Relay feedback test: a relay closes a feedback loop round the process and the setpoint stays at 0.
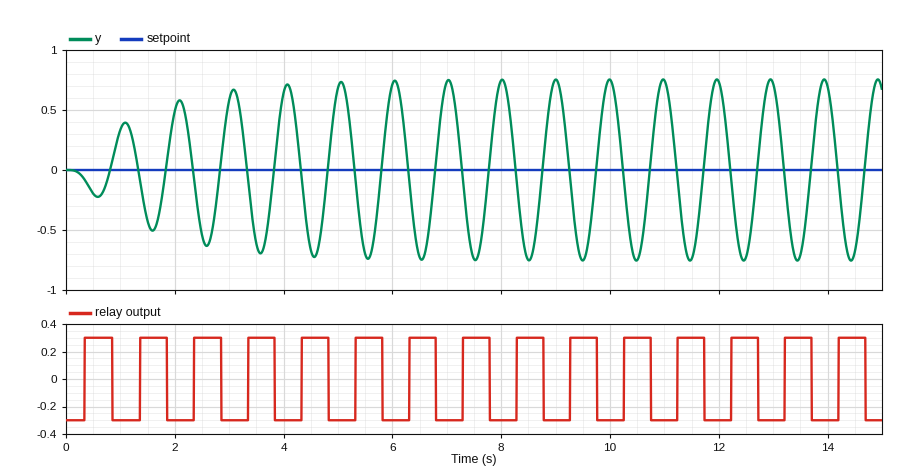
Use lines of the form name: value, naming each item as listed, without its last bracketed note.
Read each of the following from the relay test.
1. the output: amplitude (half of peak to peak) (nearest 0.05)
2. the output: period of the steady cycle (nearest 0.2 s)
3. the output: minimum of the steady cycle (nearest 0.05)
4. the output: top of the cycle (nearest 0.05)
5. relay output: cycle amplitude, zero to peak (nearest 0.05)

the output: amplitude (half of peak to peak): 0.75
the output: period of the steady cycle: 1.0 s
the output: minimum of the steady cycle: -0.75
the output: top of the cycle: 0.75
relay output: cycle amplitude, zero to peak: 0.30
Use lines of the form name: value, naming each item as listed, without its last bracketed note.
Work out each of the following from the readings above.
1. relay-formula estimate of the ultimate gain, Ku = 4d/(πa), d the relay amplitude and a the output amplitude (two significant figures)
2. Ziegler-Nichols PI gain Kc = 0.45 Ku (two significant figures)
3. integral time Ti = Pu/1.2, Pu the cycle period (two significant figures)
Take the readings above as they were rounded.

relay-formula estimate of the ultimate gain, Ku = 4d/(πa), d the relay amplitude and a the output amplitude: 0.51
Ziegler-Nichols PI gain Kc = 0.45 Ku: 0.23
integral time Ti = Pu/1.2, Pu the cycle period: 0.83 s
